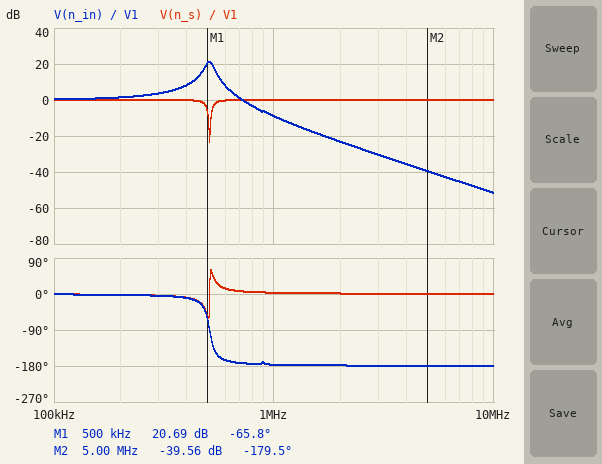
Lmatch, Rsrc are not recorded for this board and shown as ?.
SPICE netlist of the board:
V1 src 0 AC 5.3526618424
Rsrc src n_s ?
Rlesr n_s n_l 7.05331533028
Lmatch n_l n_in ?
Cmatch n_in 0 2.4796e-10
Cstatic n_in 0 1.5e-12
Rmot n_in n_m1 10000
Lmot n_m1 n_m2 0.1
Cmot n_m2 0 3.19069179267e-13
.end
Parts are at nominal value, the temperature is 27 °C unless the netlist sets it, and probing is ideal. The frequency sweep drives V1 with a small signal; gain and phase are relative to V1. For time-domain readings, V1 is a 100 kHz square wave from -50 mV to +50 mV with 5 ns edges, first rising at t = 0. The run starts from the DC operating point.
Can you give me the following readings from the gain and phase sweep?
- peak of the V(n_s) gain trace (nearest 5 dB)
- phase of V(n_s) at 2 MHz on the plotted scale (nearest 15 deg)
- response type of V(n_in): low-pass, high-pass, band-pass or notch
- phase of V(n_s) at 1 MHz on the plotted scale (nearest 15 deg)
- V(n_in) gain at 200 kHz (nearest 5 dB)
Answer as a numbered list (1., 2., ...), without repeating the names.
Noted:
1. 0 dB
2. 0 deg
3. low-pass
4. 0 deg
5. 0 dB
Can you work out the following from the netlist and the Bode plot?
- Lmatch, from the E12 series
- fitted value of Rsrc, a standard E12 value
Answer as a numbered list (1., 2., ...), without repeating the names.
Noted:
1. 390 µH
2. 100 Ω
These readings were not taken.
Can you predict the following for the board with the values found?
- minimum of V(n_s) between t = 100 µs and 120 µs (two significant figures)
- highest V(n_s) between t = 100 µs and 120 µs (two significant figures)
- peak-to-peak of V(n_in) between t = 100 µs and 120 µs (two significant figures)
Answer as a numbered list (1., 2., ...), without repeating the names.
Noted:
1. -62 mV
2. 62 mV
3. 430 mV
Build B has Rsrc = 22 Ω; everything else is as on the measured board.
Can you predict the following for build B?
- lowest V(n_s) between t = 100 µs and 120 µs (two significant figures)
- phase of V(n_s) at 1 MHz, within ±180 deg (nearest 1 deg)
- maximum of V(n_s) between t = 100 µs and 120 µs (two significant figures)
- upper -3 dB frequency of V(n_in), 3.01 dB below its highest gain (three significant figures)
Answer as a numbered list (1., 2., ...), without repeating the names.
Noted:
1. -55 mV
2. 1 deg
3. 55 mV
4. 516 kHz
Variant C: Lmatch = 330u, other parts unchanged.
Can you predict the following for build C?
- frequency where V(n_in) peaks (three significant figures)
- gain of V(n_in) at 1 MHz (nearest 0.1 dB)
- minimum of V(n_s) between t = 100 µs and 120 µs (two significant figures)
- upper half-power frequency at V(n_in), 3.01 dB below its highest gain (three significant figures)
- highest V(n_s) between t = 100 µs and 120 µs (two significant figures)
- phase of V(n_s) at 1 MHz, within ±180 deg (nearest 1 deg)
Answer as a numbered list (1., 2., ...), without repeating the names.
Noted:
1. 553 kHz
2. -7.0 dB
3. -56 mV
4. 578 kHz
5. 56 mV
6. 4 deg
